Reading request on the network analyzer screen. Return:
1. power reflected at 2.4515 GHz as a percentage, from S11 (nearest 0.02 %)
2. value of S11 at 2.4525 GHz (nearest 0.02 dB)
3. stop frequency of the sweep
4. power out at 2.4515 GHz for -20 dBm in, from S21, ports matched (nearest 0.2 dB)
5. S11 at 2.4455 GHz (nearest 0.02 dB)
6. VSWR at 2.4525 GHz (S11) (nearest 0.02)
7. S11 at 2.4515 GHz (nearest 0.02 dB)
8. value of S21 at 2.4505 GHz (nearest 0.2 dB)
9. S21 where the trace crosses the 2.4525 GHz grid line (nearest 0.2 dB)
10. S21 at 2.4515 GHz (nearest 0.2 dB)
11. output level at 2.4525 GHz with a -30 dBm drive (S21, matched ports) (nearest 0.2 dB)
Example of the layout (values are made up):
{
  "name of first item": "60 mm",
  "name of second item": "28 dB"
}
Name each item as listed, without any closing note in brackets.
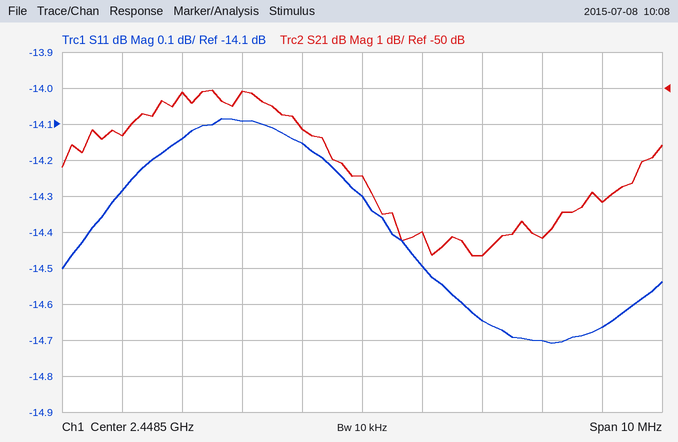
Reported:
{
  "power reflected at 2.4515 GHz as a percentage, from S11": "3.38 %",
  "value of S11 at 2.4525 GHz": "-14.66 dB",
  "stop frequency of the sweep": "2.4535 GHz",
  "power out at 2.4515 GHz for -20 dBm in, from S21, ports matched": "-74.2 dBm",
  "S11 at 2.4455 GHz": "-14.14 dB",
  "VSWR at 2.4525 GHz (S11)": "1.46",
  "S11 at 2.4515 GHz": "-14.70 dB",
  "value of S21 at 2.4505 GHz": "-54.6 dB",
  "S21 where the trace crosses the 2.4525 GHz grid line": "-53.2 dB",
  "S21 at 2.4515 GHz": "-54.2 dB",
  "output level at 2.4525 GHz with a -30 dBm drive (S21, matched ports)": "-83.2 dBm"
}
